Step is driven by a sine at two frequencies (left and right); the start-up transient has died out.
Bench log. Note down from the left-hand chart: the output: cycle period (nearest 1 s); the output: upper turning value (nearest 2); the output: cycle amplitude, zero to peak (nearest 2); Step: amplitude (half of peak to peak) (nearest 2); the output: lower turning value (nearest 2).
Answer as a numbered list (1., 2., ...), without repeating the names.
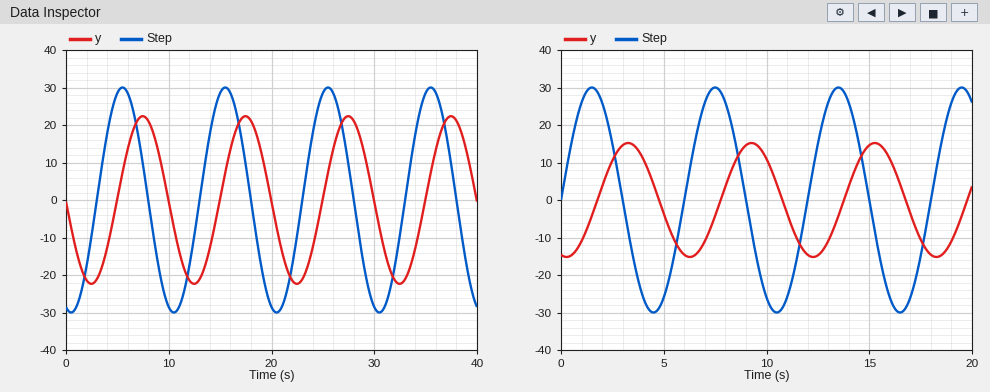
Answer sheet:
1. 10 s
2. 22
3. 22
4. 30
5. -22
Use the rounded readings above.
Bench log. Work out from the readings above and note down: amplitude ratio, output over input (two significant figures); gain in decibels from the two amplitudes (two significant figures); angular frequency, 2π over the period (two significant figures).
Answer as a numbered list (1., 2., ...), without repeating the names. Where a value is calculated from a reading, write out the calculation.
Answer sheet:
1. 22 / 30 = 0.73
2. 20 log10(22 / 30) = -2.7 dB
3. 2π / 10 = 0.63 rad/s
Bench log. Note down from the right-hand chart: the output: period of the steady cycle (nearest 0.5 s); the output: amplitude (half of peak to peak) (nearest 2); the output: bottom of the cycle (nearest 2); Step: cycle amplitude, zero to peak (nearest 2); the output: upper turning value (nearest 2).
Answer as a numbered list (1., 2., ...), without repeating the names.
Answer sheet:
1. 6.0 s
2. 16
3. -16
4. 30
5. 16
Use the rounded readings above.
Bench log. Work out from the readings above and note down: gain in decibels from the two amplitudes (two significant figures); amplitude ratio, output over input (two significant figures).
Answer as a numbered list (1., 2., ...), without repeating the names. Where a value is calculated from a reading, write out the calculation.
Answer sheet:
1. 20 log10(16 / 30) = -5.5 dB
2. 16 / 30 = 0.53
